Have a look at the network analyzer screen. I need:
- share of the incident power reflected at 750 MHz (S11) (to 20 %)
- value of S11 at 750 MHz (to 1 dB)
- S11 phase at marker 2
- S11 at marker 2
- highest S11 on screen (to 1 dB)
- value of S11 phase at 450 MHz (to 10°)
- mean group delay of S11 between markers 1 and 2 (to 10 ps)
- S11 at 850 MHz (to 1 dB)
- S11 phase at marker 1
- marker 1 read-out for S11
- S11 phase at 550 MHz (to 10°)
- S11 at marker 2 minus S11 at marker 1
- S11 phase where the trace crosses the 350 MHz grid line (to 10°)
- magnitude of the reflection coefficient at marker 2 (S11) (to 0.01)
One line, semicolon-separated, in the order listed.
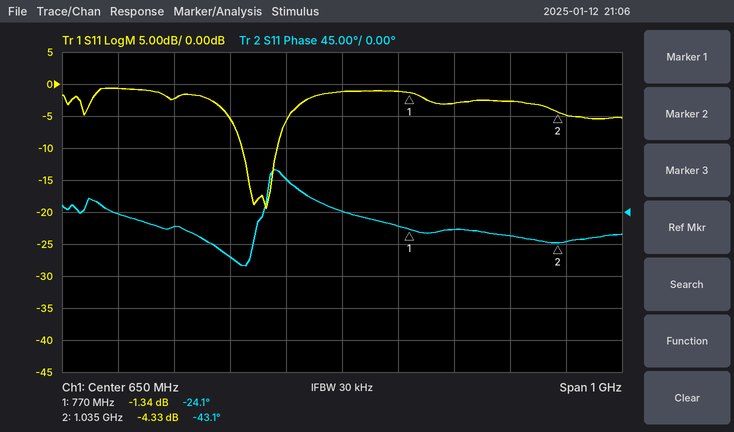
80 %; -1 dB; -43.1°; -4.33 dB; -1 dB; -60°; 200 ps; -3 dB; -24.1°; -1.34 dB; 50°; -2.99 dB; -20°; 0.61
